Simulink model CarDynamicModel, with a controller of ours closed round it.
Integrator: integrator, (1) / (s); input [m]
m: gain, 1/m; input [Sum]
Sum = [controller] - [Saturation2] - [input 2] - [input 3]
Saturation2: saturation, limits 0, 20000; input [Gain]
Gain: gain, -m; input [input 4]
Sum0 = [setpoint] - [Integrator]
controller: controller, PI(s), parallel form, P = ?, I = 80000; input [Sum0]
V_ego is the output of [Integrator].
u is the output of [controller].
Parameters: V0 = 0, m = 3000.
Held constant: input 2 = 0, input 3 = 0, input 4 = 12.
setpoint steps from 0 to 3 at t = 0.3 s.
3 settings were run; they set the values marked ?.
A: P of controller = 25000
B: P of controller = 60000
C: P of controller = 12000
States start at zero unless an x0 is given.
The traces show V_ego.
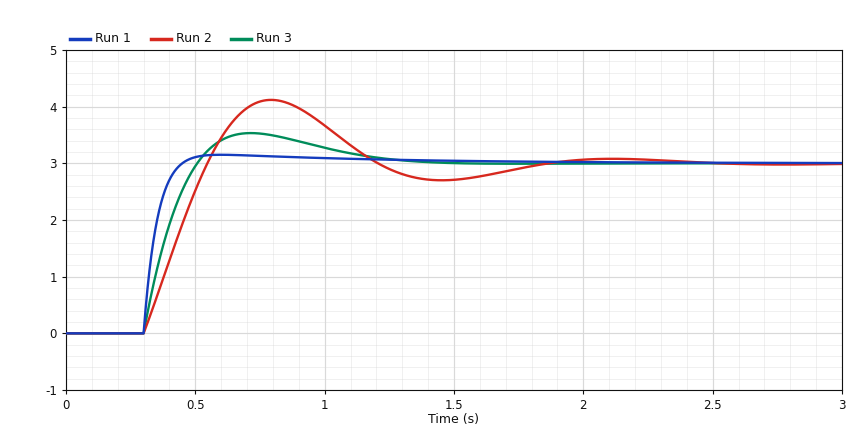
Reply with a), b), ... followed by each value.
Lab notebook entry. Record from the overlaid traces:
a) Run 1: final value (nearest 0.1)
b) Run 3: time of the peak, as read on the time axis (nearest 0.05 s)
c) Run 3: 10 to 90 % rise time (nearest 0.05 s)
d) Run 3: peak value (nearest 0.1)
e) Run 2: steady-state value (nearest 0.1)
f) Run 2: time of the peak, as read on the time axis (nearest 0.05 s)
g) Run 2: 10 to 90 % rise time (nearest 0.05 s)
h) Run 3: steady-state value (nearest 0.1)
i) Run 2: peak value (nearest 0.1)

a) 3.0
b) 0.70 s
c) 0.15 s
d) 3.5
e) 3.0
f) 0.80 s
g) 0.20 s
h) 3.0
i) 4.1
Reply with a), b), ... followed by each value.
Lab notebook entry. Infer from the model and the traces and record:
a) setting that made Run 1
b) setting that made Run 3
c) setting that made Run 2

a) B
b) A
c) C
